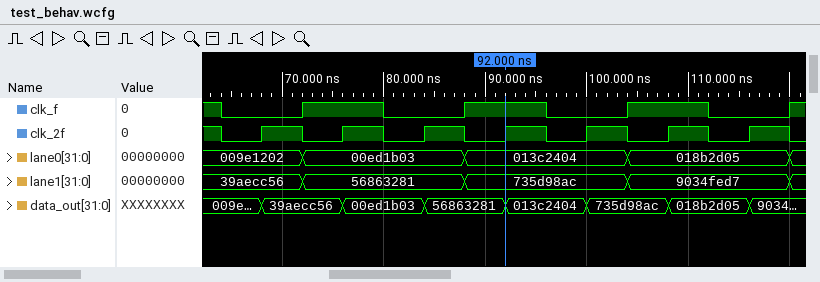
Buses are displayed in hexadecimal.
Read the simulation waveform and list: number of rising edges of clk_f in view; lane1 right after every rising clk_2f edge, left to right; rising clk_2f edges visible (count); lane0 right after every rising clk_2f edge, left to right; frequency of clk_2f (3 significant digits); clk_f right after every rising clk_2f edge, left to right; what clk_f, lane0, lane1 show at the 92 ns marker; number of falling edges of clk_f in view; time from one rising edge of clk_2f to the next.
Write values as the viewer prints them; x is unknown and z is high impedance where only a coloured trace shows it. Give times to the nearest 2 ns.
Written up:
4
39aecc56, 56863281, 56863281, 735d98ac, 735d98ac, 9034fed7, 9034fed7
7
009e1202, 00ed1b03, 00ed1b03, 013c2404, 013c2404, 018b2d05, 018b2d05
125 MHz
0 1 0 1 0 1 0
clk_f=1, lane0=013c2404, lane1=735d98ac
4
8 ns
